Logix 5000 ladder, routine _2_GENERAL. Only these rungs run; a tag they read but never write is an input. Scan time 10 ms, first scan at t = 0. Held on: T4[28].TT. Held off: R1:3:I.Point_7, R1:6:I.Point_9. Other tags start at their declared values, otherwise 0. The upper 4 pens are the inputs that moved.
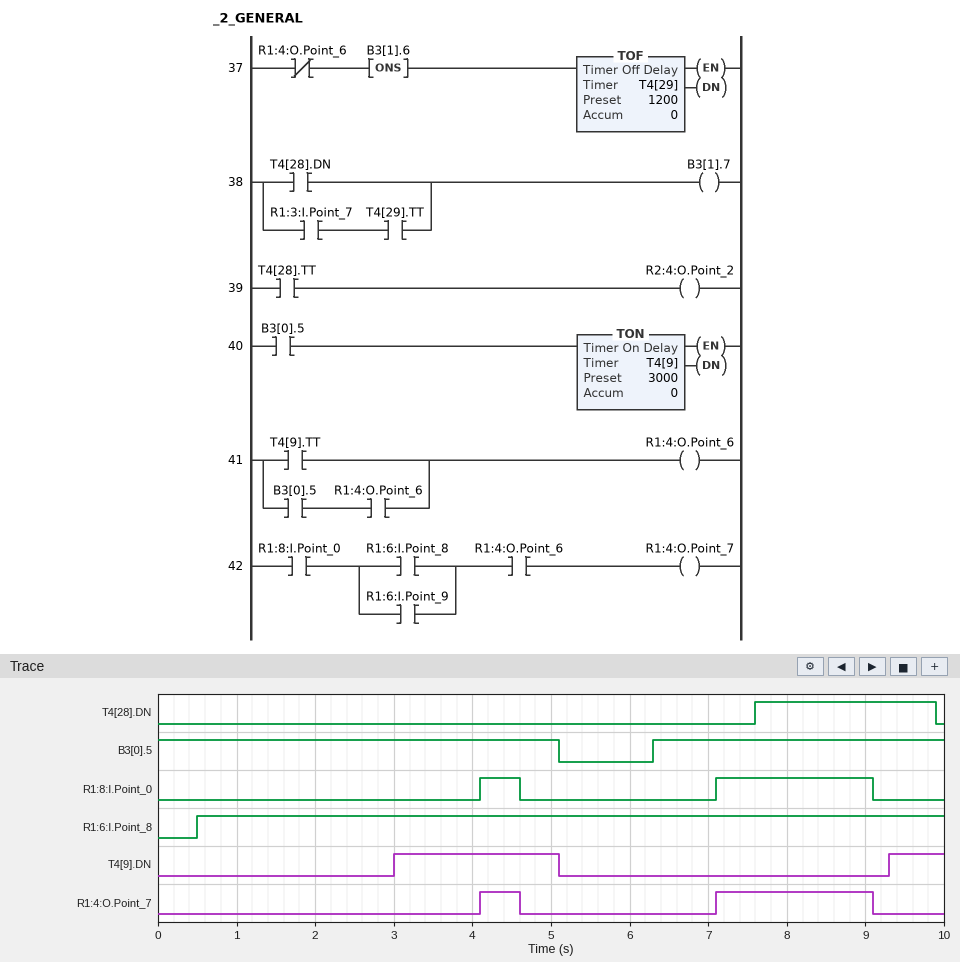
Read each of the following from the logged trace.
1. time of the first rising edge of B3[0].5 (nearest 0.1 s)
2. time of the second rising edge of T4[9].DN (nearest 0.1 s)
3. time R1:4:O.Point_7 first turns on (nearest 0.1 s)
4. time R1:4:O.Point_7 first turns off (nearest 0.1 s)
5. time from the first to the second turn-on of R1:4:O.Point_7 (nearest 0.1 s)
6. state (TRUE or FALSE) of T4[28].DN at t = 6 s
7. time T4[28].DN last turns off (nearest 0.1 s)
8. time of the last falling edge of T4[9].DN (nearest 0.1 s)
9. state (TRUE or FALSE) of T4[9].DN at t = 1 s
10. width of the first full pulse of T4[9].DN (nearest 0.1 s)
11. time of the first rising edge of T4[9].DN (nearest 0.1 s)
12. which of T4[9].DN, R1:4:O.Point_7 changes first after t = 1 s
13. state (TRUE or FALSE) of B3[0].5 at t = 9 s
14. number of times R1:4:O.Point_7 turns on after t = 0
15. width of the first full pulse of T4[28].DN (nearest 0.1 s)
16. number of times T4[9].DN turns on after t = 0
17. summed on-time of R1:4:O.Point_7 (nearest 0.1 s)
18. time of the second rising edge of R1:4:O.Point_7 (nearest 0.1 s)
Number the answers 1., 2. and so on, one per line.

1. 6.3 s
2. 9.3 s
3. 4.1 s
4. 4.6 s
5. 3.0 s
6. FALSE
7. 9.9 s
8. 5.1 s
9. FALSE
10. 2.1 s
11. 3.0 s
12. T4[9].DN
13. TRUE
14. 2
15. 2.3 s
16. 2
17. 2.5 s
18. 7.1 s
